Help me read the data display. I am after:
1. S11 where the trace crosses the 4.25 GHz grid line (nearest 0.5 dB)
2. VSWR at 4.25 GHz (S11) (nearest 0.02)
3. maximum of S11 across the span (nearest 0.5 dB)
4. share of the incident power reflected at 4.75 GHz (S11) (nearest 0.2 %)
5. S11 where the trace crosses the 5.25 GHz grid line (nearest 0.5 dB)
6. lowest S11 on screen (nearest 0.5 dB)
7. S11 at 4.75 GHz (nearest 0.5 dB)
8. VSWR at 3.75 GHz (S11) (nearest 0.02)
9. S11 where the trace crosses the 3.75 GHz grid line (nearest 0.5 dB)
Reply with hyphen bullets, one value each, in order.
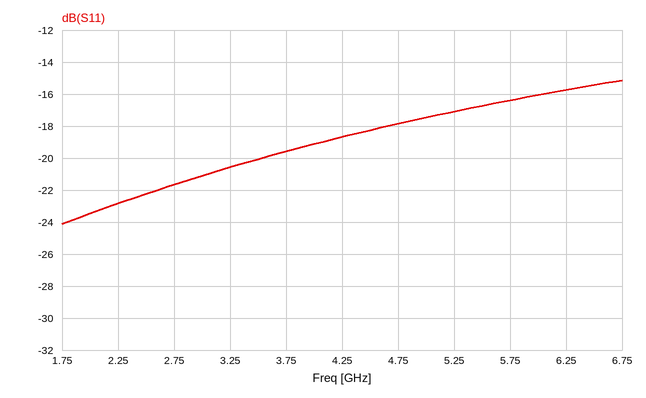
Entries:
- -18.5 dB
- 1.26
- -15.0 dB
- 1.6 %
- -17.0 dB
- -24.0 dB
- -18.0 dB
- 1.24
- -19.5 dB
